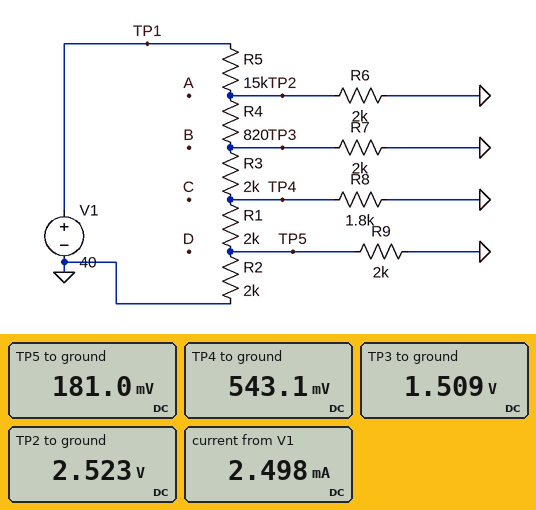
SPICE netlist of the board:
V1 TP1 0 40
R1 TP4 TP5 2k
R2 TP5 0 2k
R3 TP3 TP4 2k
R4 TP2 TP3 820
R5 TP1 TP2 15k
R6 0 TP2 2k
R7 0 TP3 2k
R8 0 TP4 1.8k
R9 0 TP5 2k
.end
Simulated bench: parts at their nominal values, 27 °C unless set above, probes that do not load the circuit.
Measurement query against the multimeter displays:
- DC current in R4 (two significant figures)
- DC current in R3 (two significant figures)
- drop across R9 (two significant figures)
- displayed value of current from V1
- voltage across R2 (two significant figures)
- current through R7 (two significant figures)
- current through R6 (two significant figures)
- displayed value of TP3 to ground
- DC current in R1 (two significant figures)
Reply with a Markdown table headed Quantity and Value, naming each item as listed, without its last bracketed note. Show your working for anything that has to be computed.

| Quantity | Value |
|---|---|
| DC current in R4 | (2.523 V - 1.509 V) / 820 Ω = 1.2 mA |
| DC current in R3 | (1.509 V - 543.1 mV) / 2 kΩ = 480 µA |
| drop across R9 | 181 mV = 180 mV |
| displayed value of current from V1 | 2.498 mA |
| voltage across R2 | 181 mV = 180 mV |
| current through R7 | (1.509 V) / 2 kΩ = 750 µA |
| current through R6 | (2.523 V) / 2 kΩ = 1.3 mA |
| displayed value of TP3 to ground | 1.509 V |
| DC current in R1 | (543.1 mV - 181 mV) / 2 kΩ = 180 µA |
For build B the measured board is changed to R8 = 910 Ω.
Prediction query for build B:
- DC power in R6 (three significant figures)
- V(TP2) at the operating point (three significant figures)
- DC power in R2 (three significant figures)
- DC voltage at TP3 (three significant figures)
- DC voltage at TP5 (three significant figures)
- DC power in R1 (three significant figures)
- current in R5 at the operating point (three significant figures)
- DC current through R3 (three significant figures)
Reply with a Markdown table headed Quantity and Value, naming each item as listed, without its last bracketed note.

| Quantity | Value |
|---|---|
| DC power in R6 | 3.08 mW |
| V(TP2) at the operating point | 2.48 V |
| DC power in R2 | 7.80 µW |
| DC voltage at TP3 | 1.45 V |
| DC voltage at TP5 | 125 mV |
| DC power in R1 | 31.2 µW |
| current in R5 at the operating point | 2.50 mA |
| DC current through R3 | 537 µA |
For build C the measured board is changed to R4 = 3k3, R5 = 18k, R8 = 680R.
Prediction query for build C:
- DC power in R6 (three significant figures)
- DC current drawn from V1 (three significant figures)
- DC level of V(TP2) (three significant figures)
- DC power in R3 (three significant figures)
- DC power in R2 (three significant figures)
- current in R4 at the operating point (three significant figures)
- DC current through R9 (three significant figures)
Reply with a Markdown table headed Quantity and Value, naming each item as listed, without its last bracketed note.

| Quantity | Value |
|---|---|
| DC power in R6 | 4.04 mW |
| DC current drawn from V1 | 2.06 mA |
| DC level of V(TP2) | 2.84 V |
| DC power in R3 | 159 µW |
| DC power in R2 | 1.36 µW |
| current in R4 at the operating point | 643 µA |
| DC current through R9 | 26.1 µA |
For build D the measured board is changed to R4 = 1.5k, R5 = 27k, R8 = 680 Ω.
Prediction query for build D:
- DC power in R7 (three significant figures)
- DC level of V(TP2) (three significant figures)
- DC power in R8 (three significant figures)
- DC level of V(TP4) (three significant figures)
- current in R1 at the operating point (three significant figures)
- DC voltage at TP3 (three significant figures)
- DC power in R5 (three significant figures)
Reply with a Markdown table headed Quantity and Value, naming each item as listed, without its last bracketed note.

| Quantity | Value |
|---|---|
| DC power in R7 | 238 µW |
| DC level of V(TP2) | 1.61 V |
| DC power in R8 | 33.0 µW |
| DC level of V(TP4) | 150 mV |
| current in R1 at the operating point | 49.9 µA |
| DC voltage at TP3 | 690 mV |
| DC power in R5 | 54.6 mW |
